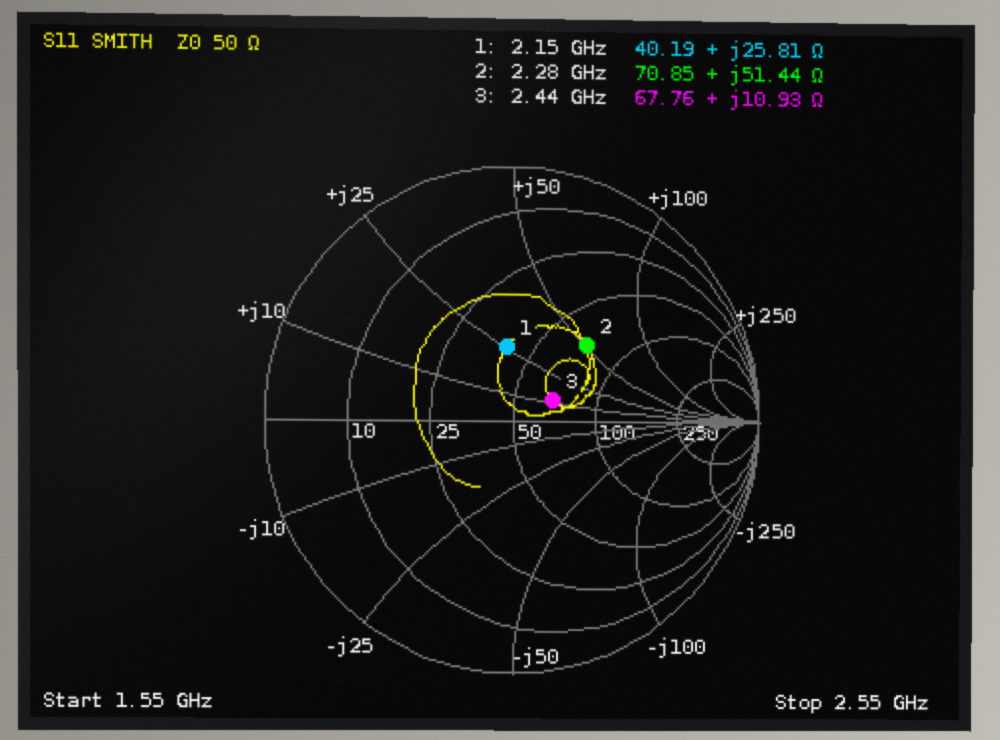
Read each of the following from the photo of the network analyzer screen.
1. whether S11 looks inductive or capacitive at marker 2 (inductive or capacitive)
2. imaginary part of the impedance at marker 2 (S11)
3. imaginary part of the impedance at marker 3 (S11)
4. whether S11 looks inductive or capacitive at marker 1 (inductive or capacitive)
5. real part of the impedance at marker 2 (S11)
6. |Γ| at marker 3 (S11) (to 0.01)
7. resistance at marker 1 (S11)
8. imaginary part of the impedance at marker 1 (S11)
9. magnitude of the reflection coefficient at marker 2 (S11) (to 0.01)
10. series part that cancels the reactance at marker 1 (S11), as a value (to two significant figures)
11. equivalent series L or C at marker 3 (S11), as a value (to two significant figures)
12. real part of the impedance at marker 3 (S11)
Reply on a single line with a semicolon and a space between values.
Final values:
inductive; +51.44 Ω; +10.93 Ω; inductive; 70.85 Ω; 0.18; 40.19 Ω; +25.81 Ω; 0.42; 2.9 pF; 710 pH; 67.76 Ω
